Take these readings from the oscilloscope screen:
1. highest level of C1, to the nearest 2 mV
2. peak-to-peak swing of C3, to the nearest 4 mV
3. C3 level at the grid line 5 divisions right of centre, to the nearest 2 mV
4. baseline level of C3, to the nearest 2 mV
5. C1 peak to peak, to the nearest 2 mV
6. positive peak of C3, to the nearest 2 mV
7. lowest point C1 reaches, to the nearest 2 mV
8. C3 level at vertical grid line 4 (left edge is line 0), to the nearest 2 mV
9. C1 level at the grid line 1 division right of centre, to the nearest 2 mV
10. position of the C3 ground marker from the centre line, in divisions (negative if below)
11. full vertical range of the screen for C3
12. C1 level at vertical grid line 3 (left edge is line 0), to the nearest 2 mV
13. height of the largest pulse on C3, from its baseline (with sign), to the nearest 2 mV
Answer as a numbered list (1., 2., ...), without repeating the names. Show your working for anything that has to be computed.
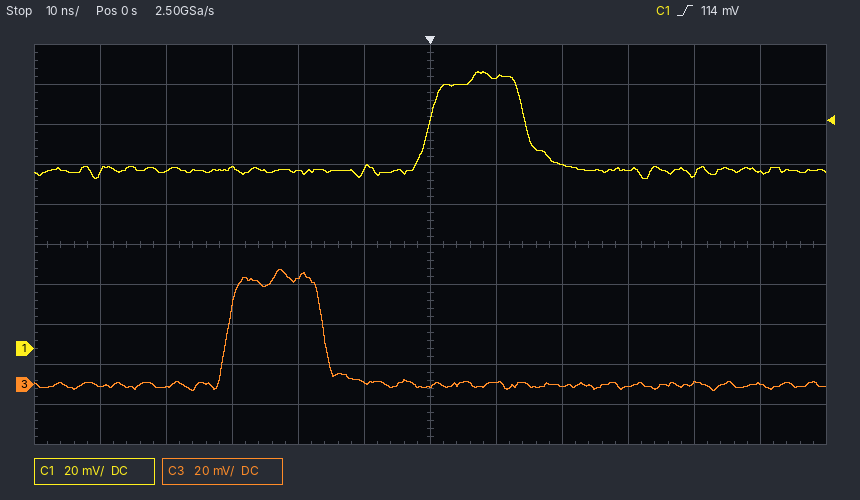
1. 138 mV
2. 60 mV
3. 0 mV
4. 0 mV
5. 138 mV − (84 mV) = 54 mV
6. 58 mV
7. 84 mV
8. 54 mV
9. 136 mV
10. -3.5 div
11. 200 mV
12. 90 mV
13. 58 mV − (0 mV) = +58 mV
